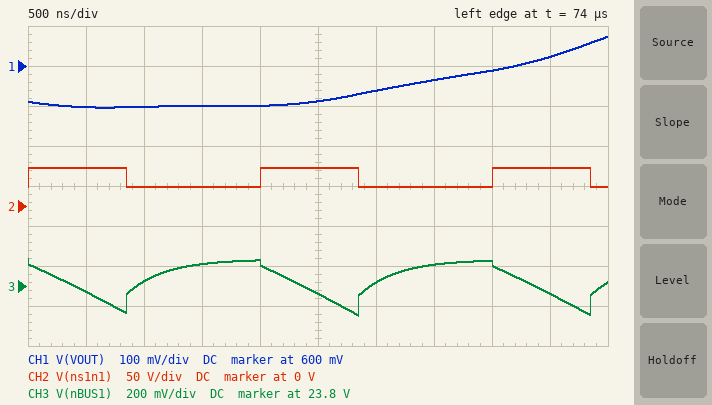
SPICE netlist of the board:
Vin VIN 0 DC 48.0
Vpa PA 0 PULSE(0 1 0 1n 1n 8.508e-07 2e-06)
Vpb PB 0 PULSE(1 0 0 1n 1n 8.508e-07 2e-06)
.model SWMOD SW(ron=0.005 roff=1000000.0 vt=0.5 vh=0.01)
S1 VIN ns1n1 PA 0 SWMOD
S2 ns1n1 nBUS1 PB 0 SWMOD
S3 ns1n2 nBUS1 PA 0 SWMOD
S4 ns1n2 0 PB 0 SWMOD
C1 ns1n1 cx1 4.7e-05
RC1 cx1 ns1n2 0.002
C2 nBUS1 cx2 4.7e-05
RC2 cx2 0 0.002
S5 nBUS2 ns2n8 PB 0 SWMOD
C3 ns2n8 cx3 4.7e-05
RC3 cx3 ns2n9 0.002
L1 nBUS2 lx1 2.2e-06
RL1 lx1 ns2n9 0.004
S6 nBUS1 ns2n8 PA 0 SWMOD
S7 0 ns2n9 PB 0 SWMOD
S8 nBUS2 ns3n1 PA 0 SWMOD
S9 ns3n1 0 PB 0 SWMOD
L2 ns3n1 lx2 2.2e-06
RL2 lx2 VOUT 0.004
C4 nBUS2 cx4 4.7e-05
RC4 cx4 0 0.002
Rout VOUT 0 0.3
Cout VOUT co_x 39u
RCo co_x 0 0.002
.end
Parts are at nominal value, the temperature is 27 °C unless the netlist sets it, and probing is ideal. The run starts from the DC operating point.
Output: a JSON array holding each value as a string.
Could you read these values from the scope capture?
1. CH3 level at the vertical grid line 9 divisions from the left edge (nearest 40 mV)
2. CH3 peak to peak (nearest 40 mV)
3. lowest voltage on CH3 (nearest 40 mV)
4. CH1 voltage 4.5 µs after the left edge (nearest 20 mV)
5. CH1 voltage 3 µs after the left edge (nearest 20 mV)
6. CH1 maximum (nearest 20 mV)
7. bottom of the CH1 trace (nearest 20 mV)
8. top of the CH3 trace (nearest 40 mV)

["23.76 V", "280 mV", "23.64 V", "620 mV", "540 mV", "680 mV", "500 mV", "23.92 V"]
